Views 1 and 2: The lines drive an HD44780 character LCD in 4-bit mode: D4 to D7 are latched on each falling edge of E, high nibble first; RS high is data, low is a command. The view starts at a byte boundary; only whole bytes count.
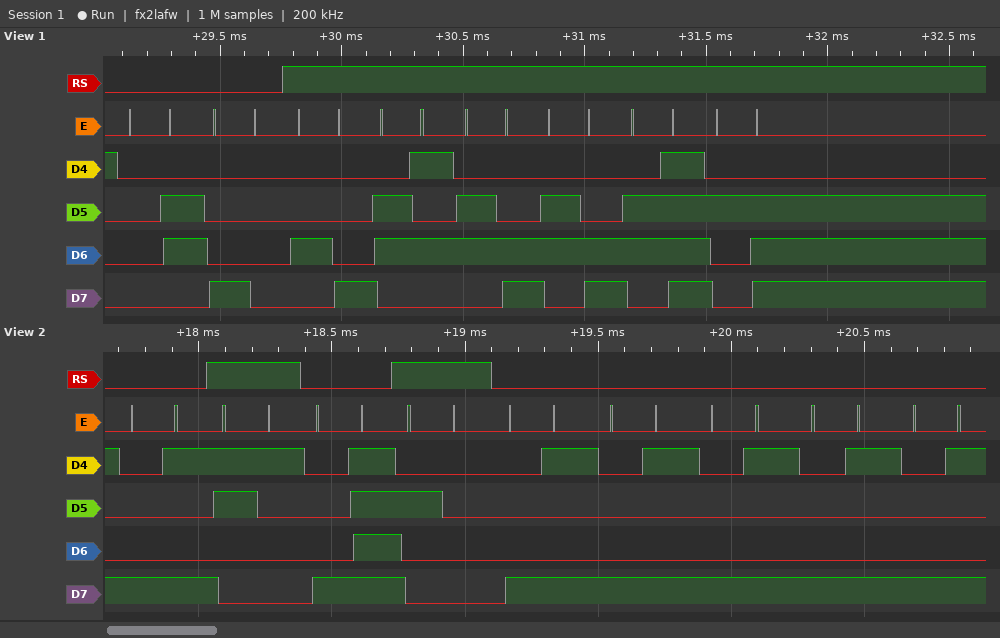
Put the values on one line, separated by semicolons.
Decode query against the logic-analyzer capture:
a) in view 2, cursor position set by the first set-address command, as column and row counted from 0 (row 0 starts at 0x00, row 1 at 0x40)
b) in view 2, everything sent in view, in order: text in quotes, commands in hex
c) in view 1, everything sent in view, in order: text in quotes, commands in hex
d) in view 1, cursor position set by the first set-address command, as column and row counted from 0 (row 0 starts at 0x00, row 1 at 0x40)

column 9, row 0; 0x89 "1" 0x8F " " 0x89 0x89 0x89 0x89 0x89; 0x06 0x80 "Hello."; column 0, row 0
